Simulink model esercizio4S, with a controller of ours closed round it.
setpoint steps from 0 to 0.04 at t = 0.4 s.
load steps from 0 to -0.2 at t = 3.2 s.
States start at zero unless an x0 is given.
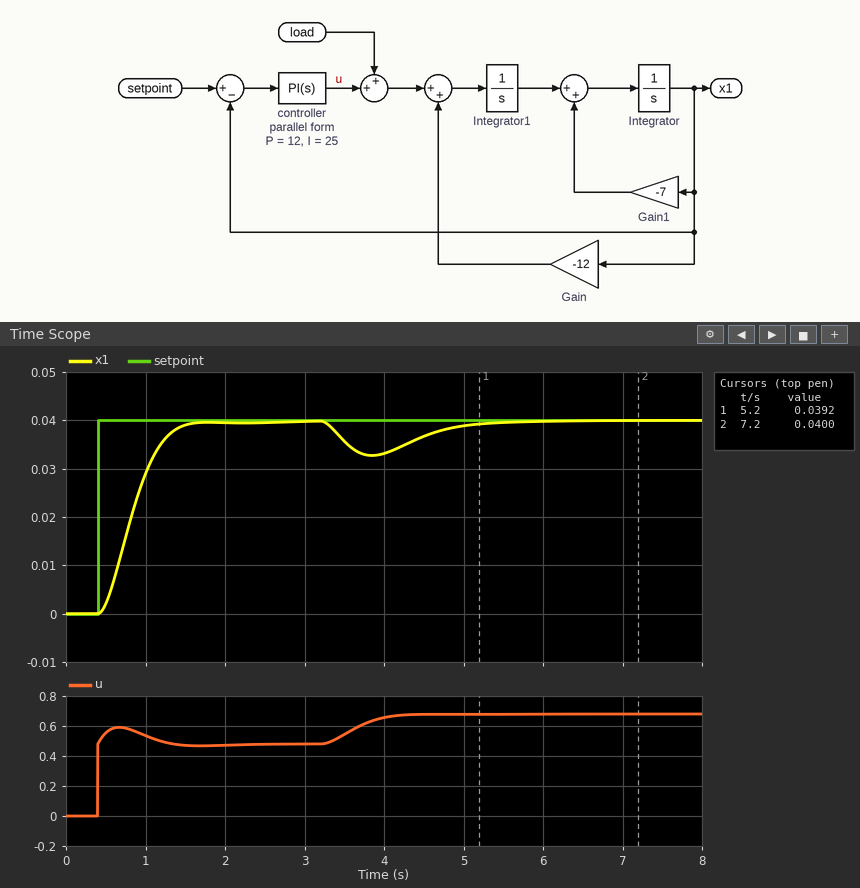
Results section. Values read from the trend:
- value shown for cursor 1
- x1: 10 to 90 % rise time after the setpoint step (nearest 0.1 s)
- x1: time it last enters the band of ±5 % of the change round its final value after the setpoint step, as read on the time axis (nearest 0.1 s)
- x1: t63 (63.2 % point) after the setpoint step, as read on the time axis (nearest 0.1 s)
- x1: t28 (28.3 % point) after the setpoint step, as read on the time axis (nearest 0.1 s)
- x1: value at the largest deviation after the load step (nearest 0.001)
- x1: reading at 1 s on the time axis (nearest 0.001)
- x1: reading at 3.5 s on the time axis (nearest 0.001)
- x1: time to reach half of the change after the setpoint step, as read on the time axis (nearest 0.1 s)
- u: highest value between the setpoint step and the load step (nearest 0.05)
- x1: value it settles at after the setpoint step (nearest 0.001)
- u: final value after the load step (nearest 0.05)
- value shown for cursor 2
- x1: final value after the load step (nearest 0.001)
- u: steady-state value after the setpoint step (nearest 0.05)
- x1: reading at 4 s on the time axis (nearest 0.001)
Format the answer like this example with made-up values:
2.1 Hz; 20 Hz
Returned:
0.0392; 0.7 s; 1.4 s; 0.9 s; 0.7 s; 0.033; 0.029; 0.036; 0.8 s; 0.60; 0.040; 0.70; 0.0400; 0.040; 0.50; 0.033
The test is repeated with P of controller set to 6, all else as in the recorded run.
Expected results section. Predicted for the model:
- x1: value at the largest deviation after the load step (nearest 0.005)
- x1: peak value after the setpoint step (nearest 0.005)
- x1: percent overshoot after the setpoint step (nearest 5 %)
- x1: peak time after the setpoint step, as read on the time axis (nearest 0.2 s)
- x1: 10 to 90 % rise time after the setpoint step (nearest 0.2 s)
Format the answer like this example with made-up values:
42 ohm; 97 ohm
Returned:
0.030; 0.045; 10 %; 2.0 s; 0.8 s
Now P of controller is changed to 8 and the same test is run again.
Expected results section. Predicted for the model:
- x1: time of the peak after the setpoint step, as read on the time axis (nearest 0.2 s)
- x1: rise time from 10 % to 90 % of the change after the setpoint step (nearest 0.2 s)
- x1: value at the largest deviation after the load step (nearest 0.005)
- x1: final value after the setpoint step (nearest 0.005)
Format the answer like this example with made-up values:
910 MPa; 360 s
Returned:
2.0 s; 0.8 s; 0.030; 0.040
